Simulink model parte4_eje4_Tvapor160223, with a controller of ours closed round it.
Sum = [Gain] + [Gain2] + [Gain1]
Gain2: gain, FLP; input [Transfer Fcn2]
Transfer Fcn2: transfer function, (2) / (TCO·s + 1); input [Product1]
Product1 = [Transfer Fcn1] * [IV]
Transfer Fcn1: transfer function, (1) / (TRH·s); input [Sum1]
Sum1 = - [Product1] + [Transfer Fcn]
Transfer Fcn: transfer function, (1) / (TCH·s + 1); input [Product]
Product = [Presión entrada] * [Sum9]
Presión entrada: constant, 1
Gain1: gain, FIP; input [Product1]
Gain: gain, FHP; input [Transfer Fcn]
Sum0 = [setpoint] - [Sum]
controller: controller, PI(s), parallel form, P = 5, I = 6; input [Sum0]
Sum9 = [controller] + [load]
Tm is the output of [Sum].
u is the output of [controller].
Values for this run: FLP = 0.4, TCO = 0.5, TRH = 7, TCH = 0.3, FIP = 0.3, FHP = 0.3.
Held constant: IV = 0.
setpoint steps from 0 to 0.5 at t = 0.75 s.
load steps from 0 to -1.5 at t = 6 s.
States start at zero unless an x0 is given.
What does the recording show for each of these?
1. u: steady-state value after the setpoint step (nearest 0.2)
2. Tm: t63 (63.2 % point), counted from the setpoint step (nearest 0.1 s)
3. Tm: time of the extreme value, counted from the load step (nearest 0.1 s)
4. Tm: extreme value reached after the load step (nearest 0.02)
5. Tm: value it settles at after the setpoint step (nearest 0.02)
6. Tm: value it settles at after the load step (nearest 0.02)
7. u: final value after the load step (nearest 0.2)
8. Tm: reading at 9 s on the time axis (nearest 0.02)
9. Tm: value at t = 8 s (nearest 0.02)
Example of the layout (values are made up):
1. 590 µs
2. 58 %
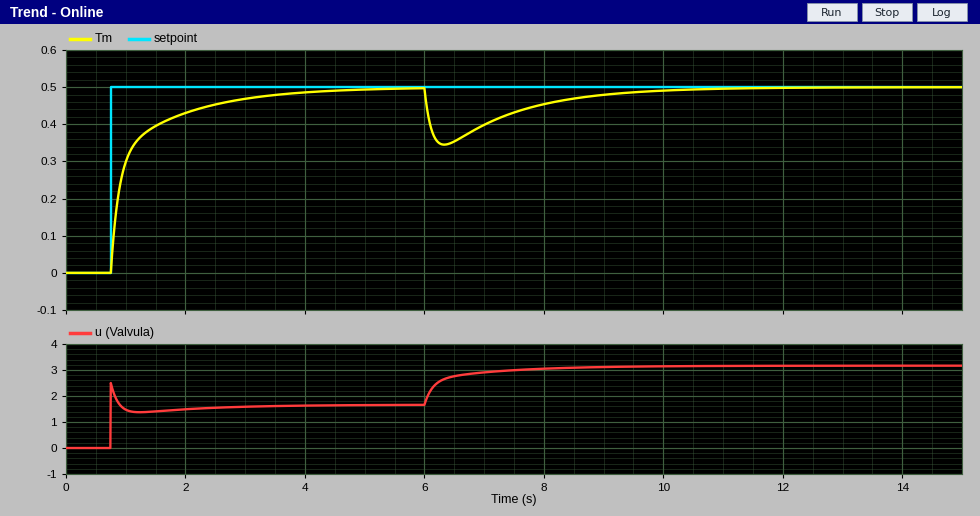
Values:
1. 1.6
2. 0.3 s
3. 0.3 s
4. 0.34
5. 0.50
6. 0.50
7. 3.2
8. 0.48
9. 0.46
